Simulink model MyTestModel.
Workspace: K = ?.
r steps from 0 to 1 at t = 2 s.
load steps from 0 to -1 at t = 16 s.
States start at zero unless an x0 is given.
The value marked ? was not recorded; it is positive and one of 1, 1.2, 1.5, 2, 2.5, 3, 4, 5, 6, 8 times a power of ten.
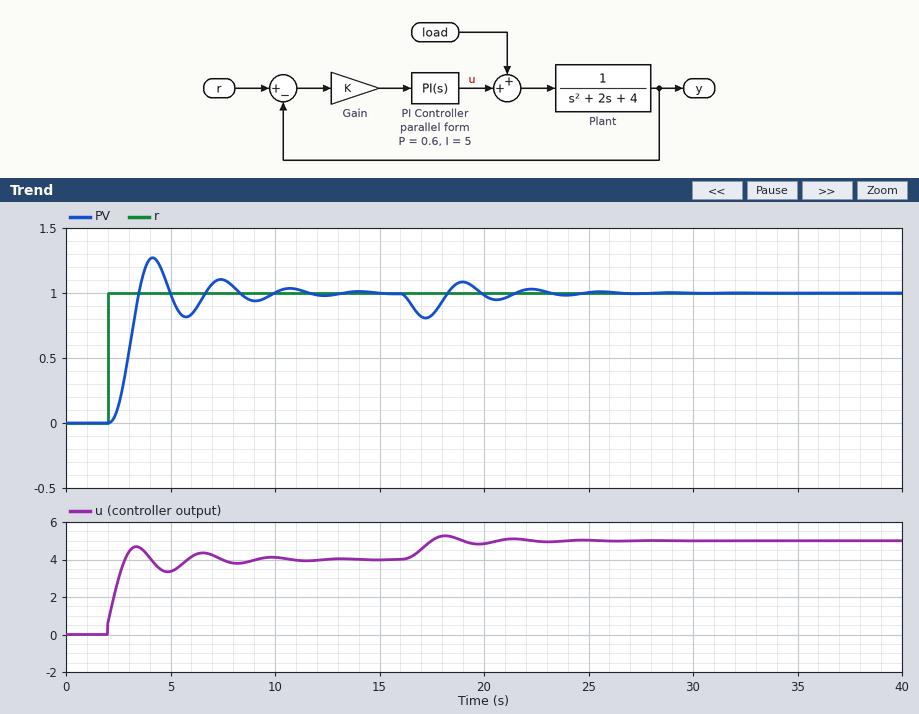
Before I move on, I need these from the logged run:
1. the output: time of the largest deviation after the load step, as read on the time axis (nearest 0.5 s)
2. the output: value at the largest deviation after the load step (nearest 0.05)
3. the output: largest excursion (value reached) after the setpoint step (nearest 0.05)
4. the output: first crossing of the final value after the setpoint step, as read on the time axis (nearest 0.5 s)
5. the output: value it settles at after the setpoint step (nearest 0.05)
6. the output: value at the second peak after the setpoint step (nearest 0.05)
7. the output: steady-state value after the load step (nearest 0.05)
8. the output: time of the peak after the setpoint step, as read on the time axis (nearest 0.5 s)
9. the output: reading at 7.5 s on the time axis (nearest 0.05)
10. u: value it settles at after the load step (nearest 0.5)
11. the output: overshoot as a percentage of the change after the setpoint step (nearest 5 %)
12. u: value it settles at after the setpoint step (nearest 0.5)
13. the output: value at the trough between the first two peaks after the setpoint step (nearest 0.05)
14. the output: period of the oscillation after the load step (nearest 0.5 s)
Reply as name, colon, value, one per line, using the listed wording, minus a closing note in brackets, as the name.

the output: time of the largest deviation after the load step, as read on the time axis: 17.0 s
the output: value at the largest deviation after the load step: 0.80
the output: largest excursion (value reached) after the setpoint step: 1.25
the output: first crossing of the final value after the setpoint step, as read on the time axis: 3.5 s
the output: value it settles at after the setpoint step: 1.00
the output: value at the second peak after the setpoint step: 1.10
the output: steady-state value after the load step: 1.00
the output: time of the peak after the setpoint step, as read on the time axis: 4.0 s
the output: reading at 7.5 s on the time axis: 1.10
u: value it settles at after the load step: 5.0
the output: overshoot as a percentage of the change after the setpoint step: 25 %
u: value it settles at after the setpoint step: 4.0
the output: value at the trough between the first two peaks after the setpoint step: 0.80
the output: period of the oscillation after the load step: 3.5 s
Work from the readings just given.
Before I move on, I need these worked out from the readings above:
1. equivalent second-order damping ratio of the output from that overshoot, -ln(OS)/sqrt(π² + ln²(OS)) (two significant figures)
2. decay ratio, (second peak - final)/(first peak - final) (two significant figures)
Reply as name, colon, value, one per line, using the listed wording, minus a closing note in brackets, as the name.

equivalent second-order damping ratio of the output from that overshoot, -ln(OS)/sqrt(π² + ln²(OS)): 0.40
decay ratio, (second peak - final)/(first peak - final): 0.40
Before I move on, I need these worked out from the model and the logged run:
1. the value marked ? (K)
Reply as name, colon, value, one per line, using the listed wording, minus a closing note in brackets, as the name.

the value marked ?: 1
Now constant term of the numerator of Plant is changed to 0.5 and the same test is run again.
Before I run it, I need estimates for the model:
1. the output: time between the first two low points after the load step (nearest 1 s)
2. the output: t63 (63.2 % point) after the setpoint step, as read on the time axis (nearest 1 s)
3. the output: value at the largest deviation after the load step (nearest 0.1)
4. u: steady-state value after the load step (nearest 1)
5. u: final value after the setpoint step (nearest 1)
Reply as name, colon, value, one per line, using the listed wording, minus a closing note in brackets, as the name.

the output: time between the first two low points after the load step: 4 s
the output: t63 (63.2 % point) after the setpoint step, as read on the time axis: 4 s
the output: value at the largest deviation after the load step: 0.9
u: steady-state value after the load step: 9
u: final value after the setpoint step: 8
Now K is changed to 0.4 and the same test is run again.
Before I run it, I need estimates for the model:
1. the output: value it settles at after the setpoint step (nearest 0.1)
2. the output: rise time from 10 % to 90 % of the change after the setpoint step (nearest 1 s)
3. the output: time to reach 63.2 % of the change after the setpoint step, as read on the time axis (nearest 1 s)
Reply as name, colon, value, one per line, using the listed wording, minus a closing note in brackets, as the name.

the output: value it settles at after the setpoint step: 1.0
the output: rise time from 10 % to 90 % of the change after the setpoint step: 4 s
the output: time to reach 63.2 % of the change after the setpoint step, as read on the time axis: 4 s
